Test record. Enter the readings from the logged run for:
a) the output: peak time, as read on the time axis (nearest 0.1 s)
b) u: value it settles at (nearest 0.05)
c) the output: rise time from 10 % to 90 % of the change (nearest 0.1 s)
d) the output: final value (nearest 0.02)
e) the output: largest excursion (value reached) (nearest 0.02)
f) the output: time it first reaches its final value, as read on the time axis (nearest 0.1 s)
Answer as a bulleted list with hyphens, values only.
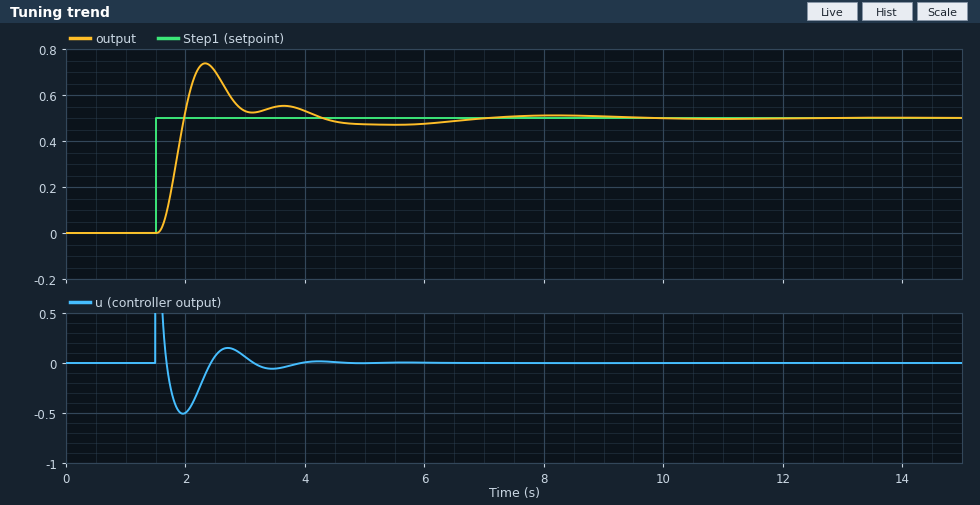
- 2.3 s
- 0.00
- 0.3 s
- 0.50
- 0.74
- 2.0 s
